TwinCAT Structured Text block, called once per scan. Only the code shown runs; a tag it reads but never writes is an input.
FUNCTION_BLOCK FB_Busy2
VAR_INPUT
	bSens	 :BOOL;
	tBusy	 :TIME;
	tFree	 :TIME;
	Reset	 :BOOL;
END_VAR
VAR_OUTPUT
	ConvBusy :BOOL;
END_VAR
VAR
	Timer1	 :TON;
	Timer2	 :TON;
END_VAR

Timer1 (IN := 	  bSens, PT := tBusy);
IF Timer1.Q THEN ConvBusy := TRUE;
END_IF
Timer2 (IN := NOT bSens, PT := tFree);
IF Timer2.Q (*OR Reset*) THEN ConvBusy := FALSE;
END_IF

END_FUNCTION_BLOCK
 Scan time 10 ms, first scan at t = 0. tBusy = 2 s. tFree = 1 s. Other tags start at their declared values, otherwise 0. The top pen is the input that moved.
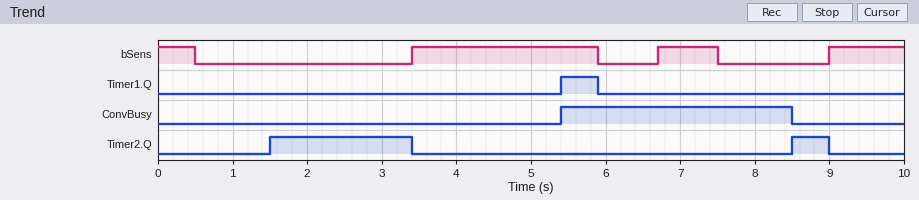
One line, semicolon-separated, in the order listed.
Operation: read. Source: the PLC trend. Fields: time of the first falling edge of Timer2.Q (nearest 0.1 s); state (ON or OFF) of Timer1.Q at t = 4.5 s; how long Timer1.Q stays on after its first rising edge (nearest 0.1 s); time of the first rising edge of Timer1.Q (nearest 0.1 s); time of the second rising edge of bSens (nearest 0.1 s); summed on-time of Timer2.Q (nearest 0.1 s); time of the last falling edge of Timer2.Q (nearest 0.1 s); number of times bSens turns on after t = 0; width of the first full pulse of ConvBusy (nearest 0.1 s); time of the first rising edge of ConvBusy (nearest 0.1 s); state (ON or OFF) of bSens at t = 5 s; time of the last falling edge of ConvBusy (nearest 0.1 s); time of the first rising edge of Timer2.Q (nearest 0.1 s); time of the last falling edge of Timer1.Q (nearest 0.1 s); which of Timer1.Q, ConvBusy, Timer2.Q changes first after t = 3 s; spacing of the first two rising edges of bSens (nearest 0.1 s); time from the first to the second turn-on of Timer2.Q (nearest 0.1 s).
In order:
3.4 s; OFF; 0.5 s; 5.4 s; 6.7 s; 2.4 s; 9.0 s; 3; 3.1 s; 5.4 s; ON; 8.5 s; 1.5 s; 5.9 s; Timer2.Q; 3.3 s; 7.0 s
